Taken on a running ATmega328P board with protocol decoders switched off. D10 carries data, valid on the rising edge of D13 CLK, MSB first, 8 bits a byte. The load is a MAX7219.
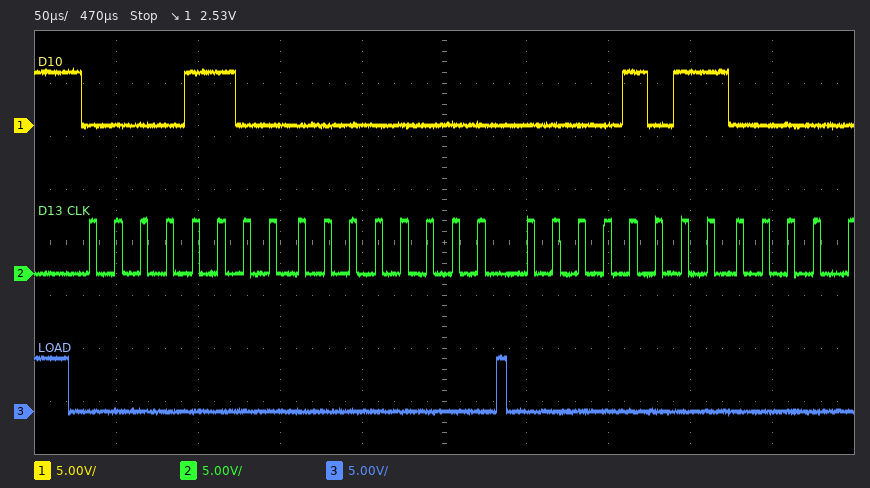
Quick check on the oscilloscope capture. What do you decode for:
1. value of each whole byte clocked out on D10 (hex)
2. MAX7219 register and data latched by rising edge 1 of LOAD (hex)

0x0C 0x00 0x0B
register 0xC, data 0x00
